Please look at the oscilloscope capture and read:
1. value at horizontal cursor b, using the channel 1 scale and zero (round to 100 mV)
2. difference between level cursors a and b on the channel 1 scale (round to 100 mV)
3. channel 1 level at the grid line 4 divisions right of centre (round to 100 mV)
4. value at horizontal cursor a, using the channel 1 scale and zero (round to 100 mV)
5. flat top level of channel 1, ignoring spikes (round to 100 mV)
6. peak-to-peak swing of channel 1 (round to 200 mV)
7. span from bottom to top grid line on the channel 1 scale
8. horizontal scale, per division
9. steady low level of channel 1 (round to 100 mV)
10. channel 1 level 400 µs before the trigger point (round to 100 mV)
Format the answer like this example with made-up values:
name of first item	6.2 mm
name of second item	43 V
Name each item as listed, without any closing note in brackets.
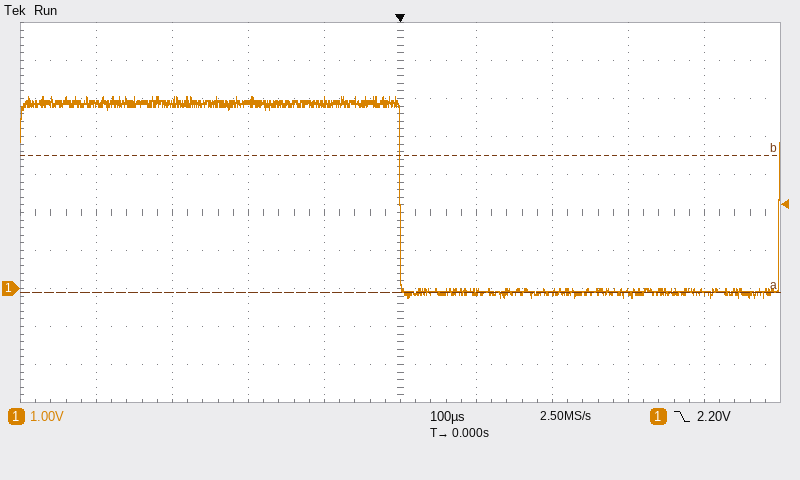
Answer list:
value at horizontal cursor b, using the channel 1 scale and zero	3.5 V
difference between level cursors a and b on the channel 1 scale	3.6 V
channel 1 level at the grid line 4 divisions right of centre	-100 mV
value at horizontal cursor a, using the channel 1 scale and zero	-100 mV
flat top level of channel 1, ignoring spikes	4.9 V
peak-to-peak swing of channel 1	5.2 V
span from bottom to top grid line on the channel 1 scale	10 V
horizontal scale, per division	100 µs
steady low level of channel 1	-100 mV
channel 1 level 400 µs before the trigger point	4.9 V
